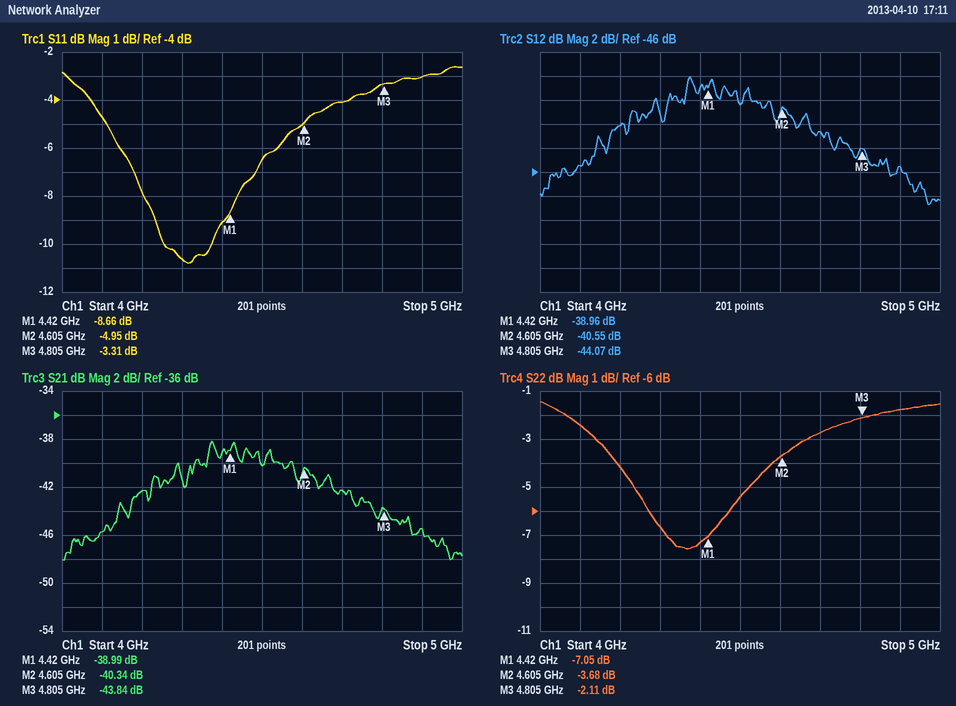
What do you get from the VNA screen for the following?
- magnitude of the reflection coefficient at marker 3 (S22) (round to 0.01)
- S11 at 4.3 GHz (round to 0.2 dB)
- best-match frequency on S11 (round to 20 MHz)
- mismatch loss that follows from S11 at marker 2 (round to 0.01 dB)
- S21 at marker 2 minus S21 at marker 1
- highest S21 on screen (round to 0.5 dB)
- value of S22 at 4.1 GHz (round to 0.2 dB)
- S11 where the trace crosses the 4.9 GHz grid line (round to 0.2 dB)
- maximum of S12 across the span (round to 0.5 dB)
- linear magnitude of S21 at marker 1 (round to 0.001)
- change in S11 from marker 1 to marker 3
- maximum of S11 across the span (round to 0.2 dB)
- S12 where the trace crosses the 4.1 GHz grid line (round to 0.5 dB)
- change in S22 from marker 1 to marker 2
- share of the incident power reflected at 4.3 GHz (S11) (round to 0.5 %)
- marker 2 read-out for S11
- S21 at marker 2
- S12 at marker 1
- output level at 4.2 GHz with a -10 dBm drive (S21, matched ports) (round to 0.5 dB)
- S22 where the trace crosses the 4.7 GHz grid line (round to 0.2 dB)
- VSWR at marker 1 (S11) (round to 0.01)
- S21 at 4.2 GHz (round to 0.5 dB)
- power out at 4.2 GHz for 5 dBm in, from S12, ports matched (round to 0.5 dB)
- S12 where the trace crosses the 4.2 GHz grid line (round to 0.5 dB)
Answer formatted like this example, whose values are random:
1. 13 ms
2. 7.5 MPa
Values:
1. 0.78
2. -10.6 dB
3. 4.32 GHz
4. 1.67 dB
5. -1.35 dB
6. -38.0 dB
7. -2.4 dB
8. -3.0 dB
9. -38.0 dB
10. 0.011
11. 5.35 dB
12. -2.6 dB
13. -45.5 dB
14. 3.37 dB
15. 8.5 %
16. -4.95 dB
17. -40.34 dB
18. -38.96 dB
19. -52.5 dBm
20. -2.8 dB
21. 2.17
22. -42.5 dB
23. -37.0 dBm
24. -42.0 dB
